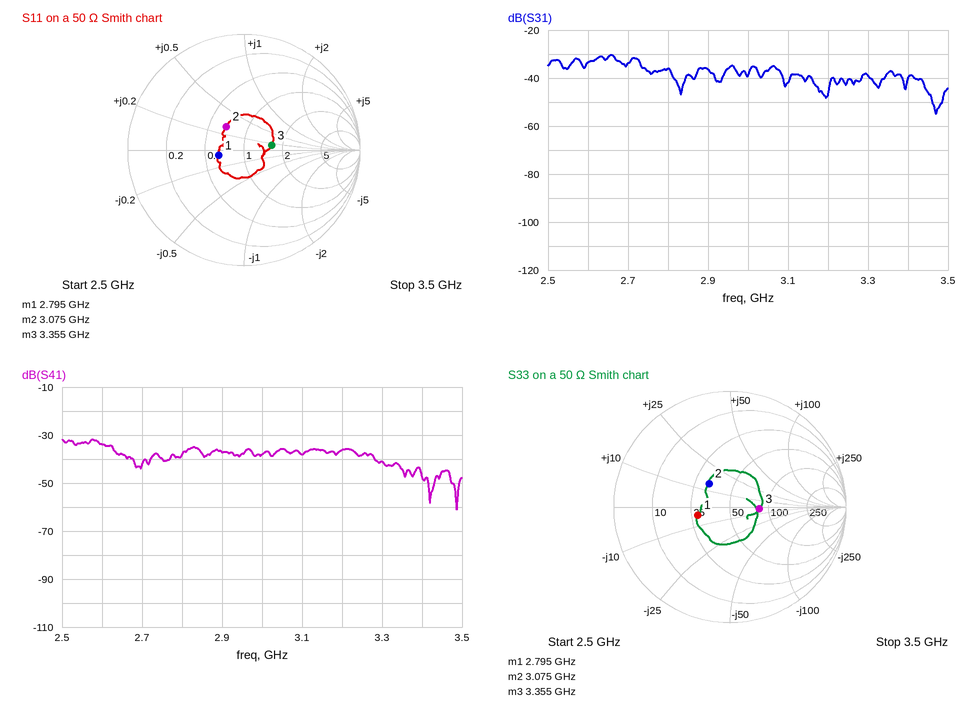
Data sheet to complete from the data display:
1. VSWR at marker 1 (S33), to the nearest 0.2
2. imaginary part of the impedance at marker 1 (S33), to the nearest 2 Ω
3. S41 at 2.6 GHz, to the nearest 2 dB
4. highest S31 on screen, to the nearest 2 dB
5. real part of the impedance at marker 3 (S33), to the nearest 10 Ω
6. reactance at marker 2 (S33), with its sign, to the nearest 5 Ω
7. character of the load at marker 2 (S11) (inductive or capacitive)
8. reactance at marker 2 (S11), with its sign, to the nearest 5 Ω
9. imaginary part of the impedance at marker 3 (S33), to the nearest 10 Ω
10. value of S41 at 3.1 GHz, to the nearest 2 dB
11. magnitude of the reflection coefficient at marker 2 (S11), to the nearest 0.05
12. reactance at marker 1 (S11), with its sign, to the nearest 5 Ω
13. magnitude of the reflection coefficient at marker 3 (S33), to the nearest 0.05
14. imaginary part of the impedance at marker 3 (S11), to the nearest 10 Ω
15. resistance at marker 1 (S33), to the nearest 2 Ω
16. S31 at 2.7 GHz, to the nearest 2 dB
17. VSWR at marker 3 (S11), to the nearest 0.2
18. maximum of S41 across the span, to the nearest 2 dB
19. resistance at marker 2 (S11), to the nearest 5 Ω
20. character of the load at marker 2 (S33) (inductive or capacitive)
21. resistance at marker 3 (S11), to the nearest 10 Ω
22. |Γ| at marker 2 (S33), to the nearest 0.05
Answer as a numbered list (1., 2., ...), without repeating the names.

1. 1.8
2. -4 Ω
3. -34 dB
4. -30 dB
5. 80 Ω
6. +15 Ω
7. inductive
8. +15 Ω
9. 0 Ω
10. -38 dB
11. 0.25
12. -5 Ω
13. 0.25
14. +10 Ω
15. 28 Ω
16. -34 dB
17. 1.6
18. -32 dB
19. 35 Ω
20. inductive
21. 80 Ω
22. 0.25
